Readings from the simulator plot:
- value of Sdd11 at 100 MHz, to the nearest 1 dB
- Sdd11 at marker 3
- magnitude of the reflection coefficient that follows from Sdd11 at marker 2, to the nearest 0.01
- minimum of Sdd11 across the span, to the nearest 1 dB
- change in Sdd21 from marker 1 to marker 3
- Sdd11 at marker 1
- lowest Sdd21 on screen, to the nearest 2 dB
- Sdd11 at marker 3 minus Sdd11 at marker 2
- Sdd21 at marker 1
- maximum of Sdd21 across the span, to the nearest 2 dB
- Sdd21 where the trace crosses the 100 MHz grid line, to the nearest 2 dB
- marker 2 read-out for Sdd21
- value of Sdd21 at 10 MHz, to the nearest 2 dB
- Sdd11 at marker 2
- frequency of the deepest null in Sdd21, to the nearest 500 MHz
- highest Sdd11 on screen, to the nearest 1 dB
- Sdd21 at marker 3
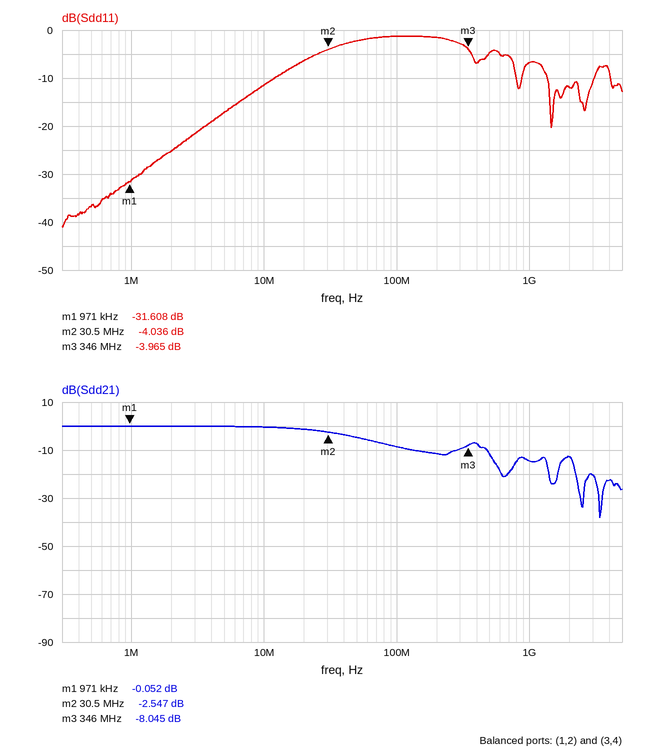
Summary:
-1 dB
-3.965 dB
0.63
-41 dB
-7.993 dB
-31.608 dB
-38 dB
0.071 dB
-0.052 dB
0 dB
-8 dB
-2.547 dB
0 dB
-4.036 dB
3.5 GHz
-1 dB
-8.045 dB
